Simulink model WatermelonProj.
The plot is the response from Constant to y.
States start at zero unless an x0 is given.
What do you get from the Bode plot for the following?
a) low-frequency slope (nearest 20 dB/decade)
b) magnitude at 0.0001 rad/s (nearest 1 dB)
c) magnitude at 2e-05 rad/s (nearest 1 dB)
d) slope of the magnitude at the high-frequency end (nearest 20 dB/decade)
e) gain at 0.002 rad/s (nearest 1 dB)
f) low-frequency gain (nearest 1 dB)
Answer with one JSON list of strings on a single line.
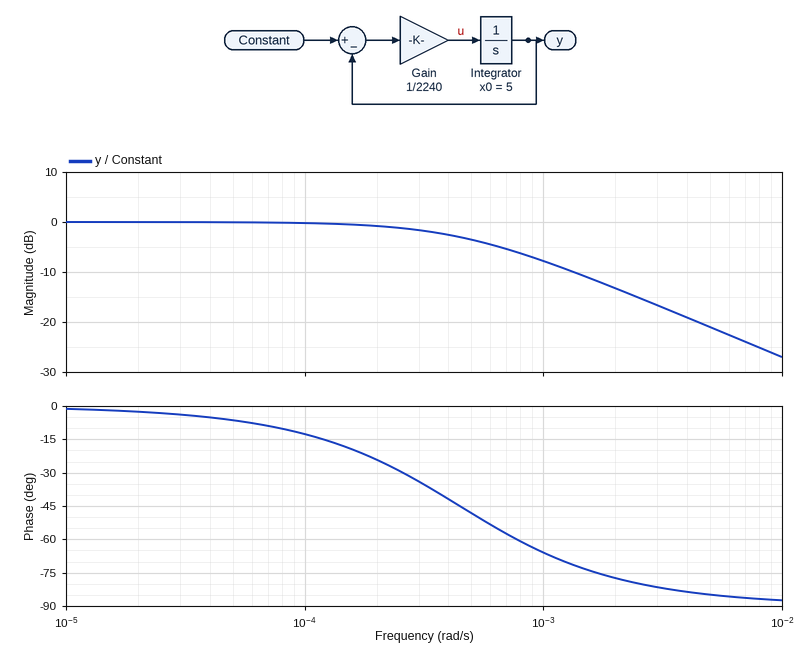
["0 dB/decade", "0 dB", "0 dB", "-20 dB/decade", "-13 dB", "0 dB"]
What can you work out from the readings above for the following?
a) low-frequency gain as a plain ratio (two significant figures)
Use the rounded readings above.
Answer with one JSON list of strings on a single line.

["1.0"]
